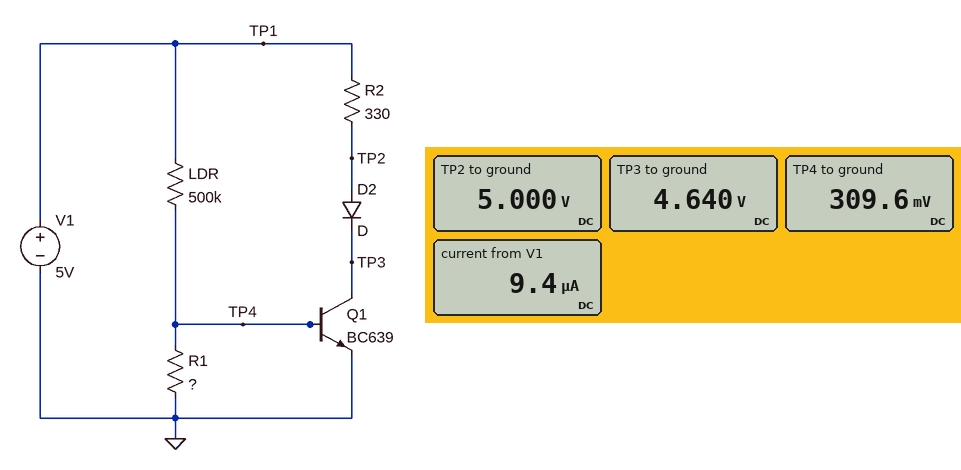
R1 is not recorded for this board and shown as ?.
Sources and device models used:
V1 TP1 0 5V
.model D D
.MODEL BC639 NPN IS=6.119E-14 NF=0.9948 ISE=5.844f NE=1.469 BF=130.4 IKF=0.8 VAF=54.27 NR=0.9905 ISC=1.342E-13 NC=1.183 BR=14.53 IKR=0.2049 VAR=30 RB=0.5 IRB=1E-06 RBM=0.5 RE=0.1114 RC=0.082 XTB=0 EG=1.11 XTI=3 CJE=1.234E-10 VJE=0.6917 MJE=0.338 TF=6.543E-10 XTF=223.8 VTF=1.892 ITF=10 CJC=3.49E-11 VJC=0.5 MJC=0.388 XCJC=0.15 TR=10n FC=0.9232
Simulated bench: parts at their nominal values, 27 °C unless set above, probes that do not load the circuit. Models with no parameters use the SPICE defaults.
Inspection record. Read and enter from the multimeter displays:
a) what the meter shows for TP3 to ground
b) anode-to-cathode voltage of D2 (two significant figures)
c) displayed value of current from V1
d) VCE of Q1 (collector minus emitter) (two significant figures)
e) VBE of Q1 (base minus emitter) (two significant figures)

4.640 V
360 mV
9.4 µA
4.6 V
310 mV
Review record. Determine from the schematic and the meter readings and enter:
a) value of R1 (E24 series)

33 kΩ
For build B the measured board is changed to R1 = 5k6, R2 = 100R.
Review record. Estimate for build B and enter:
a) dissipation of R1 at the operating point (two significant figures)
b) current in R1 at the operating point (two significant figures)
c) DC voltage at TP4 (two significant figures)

550 nW
9.9 µA
55 mV
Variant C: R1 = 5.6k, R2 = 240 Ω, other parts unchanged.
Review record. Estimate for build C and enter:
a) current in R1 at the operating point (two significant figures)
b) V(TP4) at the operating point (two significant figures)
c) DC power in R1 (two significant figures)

9.9 µA
55 mV
550 nW
